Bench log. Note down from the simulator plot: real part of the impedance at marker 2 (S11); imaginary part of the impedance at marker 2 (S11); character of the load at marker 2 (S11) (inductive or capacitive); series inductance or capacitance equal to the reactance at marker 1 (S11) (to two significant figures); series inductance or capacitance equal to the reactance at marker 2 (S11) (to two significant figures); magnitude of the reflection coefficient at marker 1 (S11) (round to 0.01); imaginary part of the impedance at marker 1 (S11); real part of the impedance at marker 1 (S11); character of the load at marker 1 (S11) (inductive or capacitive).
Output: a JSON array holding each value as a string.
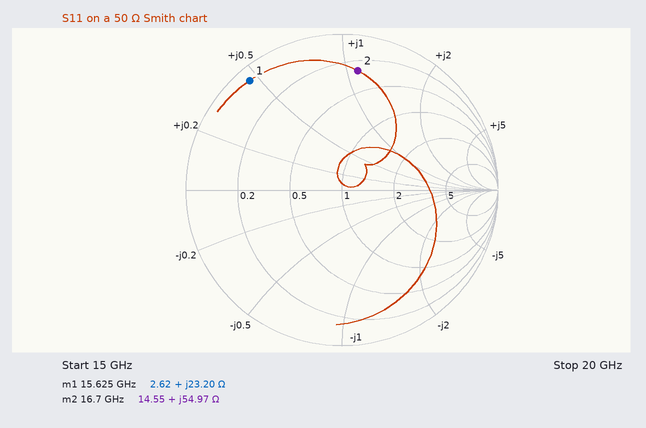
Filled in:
["14.55 Ω", "+54.97 Ω", "inductive", "240 pH", "520 pH", "0.92", "+23.20 Ω", "2.62 Ω", "inductive"]
